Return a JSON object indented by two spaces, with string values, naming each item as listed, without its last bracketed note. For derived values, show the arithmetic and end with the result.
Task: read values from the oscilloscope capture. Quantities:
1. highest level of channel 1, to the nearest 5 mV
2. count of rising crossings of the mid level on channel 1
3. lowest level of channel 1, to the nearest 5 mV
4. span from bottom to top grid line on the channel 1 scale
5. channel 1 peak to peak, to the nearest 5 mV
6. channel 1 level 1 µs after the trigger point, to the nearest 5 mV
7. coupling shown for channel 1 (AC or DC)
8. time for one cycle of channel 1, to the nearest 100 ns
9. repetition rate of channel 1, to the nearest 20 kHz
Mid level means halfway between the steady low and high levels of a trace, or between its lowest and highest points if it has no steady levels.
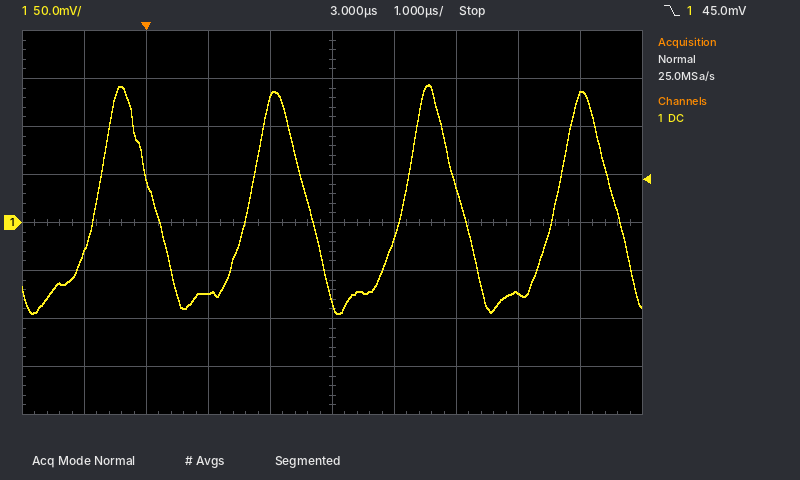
{
  "highest level of channel 1, to the nearest 5 mV": "145 mV",
  "count of rising crossings of the mid level on channel 1": "4",
  "lowest level of channel 1, to the nearest 5 mV": "-95 mV",
  "span from bottom to top grid line on the channel 1 scale": "400 mV",
  "channel 1 peak to peak, to the nearest 5 mV": "145 mV − (-95 mV) = 240 mV",
  "channel 1 level 1 µs after the trigger point, to the nearest 5 mV": "-75 mV",
  "coupling shown for channel 1": "DC",
  "time for one cycle of channel 1, to the nearest 100 ns": "2.5 µs",
  "repetition rate of channel 1, to the nearest 20 kHz": "1 / 2.5 µs ≈ 400 kHz"
}
